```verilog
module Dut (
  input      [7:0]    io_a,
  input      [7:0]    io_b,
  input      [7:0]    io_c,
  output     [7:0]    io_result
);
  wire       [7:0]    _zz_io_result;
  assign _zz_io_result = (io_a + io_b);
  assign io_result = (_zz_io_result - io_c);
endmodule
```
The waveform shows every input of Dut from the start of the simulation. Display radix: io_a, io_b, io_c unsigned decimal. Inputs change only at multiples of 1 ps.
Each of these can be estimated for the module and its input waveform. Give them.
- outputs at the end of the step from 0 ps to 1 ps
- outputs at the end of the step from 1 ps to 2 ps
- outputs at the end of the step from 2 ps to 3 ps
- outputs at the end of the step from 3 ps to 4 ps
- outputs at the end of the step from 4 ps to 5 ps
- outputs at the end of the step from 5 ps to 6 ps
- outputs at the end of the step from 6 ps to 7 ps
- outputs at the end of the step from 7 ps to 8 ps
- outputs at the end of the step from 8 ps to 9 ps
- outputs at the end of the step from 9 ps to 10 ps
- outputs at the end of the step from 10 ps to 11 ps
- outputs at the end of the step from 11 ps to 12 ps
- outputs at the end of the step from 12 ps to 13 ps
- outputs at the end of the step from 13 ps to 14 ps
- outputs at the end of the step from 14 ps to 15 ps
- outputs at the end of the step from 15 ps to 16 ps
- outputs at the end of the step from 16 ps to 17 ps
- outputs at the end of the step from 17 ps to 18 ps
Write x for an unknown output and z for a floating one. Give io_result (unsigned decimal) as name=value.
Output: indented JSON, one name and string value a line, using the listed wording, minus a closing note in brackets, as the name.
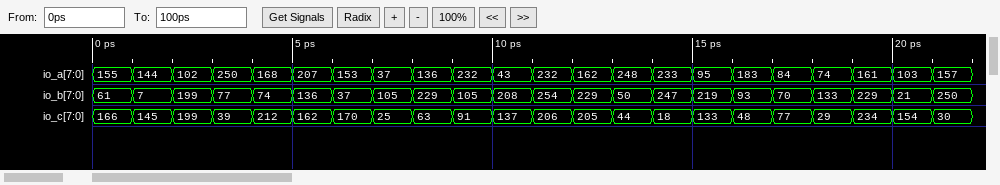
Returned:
{
  "outputs at the end of the step from 0 ps to 1 ps": "io_result=50",
  "outputs at the end of the step from 1 ps to 2 ps": "io_result=6",
  "outputs at the end of the step from 2 ps to 3 ps": "io_result=102",
  "outputs at the end of the step from 3 ps to 4 ps": "io_result=32",
  "outputs at the end of the step from 4 ps to 5 ps": "io_result=30",
  "outputs at the end of the step from 5 ps to 6 ps": "io_result=181",
  "outputs at the end of the step from 6 ps to 7 ps": "io_result=20",
  "outputs at the end of the step from 7 ps to 8 ps": "io_result=117",
  "outputs at the end of the step from 8 ps to 9 ps": "io_result=46",
  "outputs at the end of the step from 9 ps to 10 ps": "io_result=246",
  "outputs at the end of the step from 10 ps to 11 ps": "io_result=114",
  "outputs at the end of the step from 11 ps to 12 ps": "io_result=24",
  "outputs at the end of the step from 12 ps to 13 ps": "io_result=186",
  "outputs at the end of the step from 13 ps to 14 ps": "io_result=254",
  "outputs at the end of the step from 14 ps to 15 ps": "io_result=206",
  "outputs at the end of the step from 15 ps to 16 ps": "io_result=181",
  "outputs at the end of the step from 16 ps to 17 ps": "io_result=228",
  "outputs at the end of the step from 17 ps to 18 ps": "io_result=77"
}
